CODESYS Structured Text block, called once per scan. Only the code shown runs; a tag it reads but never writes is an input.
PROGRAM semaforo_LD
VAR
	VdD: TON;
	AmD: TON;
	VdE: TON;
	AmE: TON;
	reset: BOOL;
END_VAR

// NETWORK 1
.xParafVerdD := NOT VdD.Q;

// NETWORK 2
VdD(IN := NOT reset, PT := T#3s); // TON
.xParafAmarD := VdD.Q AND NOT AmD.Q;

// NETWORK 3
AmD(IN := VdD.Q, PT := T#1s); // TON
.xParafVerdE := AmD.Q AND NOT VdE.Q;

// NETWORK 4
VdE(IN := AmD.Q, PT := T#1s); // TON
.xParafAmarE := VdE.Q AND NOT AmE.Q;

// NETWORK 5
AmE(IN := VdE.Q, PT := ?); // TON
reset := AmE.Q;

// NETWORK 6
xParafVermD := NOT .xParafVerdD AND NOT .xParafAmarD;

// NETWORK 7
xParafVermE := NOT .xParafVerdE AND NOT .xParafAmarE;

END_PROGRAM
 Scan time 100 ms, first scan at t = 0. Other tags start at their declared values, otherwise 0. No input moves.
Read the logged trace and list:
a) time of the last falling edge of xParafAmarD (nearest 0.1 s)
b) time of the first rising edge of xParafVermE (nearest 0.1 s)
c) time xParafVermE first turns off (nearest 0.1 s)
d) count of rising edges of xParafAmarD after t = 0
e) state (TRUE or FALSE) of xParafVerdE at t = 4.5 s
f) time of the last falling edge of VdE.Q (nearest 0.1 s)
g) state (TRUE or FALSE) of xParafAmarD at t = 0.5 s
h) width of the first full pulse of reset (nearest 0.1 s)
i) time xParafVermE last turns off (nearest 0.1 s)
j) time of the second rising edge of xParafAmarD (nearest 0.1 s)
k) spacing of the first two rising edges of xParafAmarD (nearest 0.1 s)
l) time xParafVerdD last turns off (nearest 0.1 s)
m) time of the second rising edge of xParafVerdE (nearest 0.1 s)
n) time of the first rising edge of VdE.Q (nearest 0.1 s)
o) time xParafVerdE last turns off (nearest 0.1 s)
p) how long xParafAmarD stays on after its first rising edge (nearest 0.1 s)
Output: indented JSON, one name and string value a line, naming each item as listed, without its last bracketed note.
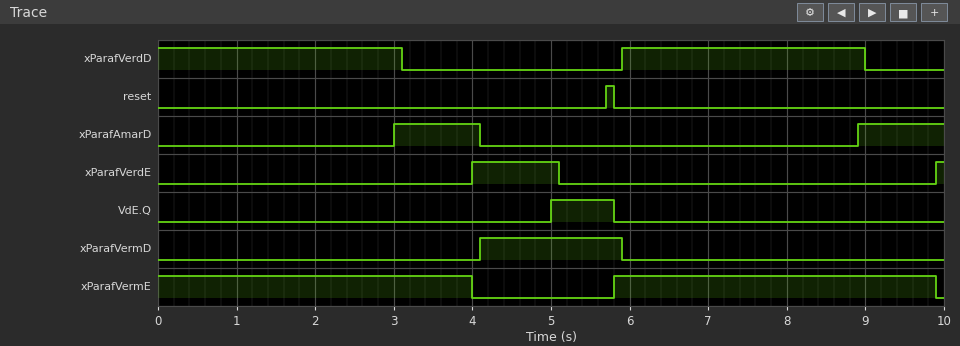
{
  "time of the last falling edge of xParafAmarD": "4.1 s",
  "time of the first rising edge of xParafVermE": "5.8 s",
  "time xParafVermE first turns off": "4.0 s",
  "count of rising edges of xParafAmarD after t = 0": "2",
  "state (TRUE or FALSE) of xParafVerdE at t = 4.5 s": "TRUE",
  "time of the last falling edge of VdE.Q": "5.8 s",
  "state (TRUE or FALSE) of xParafAmarD at t = 0.5 s": "FALSE",
  "width of the first full pulse of reset": "0.1 s",
  "time xParafVermE last turns off": "9.9 s",
  "time of the second rising edge of xParafAmarD": "8.9 s",
  "spacing of the first two rising edges of xParafAmarD": "5.9 s",
  "time xParafVerdD last turns off": "9.0 s",
  "time of the second rising edge of xParafVerdE": "9.9 s",
  "time of the first rising edge of VdE.Q": "5.0 s",
  "time xParafVerdE last turns off": "5.1 s",
  "how long xParafAmarD stays on after its first rising edge": "1.1 s"
}
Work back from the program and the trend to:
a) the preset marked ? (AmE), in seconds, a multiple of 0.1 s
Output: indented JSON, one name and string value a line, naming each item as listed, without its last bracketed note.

{
  "the preset marked ? (AmE), in seconds, a multiple of 0.1 s": "0.7 s"
}
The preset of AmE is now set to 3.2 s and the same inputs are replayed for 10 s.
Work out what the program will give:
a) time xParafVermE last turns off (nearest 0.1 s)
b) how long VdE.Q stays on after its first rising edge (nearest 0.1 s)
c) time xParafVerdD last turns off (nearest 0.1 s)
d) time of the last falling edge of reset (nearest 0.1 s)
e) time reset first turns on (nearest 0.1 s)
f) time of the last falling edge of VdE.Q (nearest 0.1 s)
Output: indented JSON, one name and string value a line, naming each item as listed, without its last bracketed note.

{
  "time xParafVermE last turns off": "4.0 s",
  "how long VdE.Q stays on after its first rising edge": "3.3 s",
  "time xParafVerdD last turns off": "3.1 s",
  "time of the last falling edge of reset": "8.3 s",
  "time reset first turns on": "8.2 s",
  "time of the last falling edge of VdE.Q": "8.3 s"
}
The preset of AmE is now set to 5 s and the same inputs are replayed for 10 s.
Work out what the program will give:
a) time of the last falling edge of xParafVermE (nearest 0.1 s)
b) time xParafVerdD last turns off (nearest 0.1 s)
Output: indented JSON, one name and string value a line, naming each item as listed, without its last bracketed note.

{
  "time of the last falling edge of xParafVermE": "4.0 s",
  "time xParafVerdD last turns off": "3.1 s"
}
